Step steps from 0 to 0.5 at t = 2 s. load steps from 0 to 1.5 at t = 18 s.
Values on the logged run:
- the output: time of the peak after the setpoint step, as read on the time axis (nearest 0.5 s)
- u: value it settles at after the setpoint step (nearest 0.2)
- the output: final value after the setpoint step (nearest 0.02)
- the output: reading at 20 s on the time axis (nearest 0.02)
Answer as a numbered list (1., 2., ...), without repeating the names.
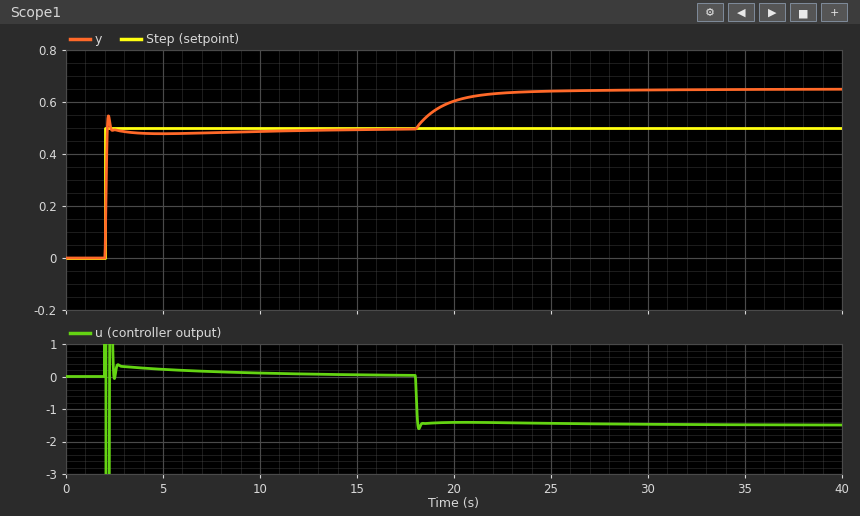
1. 2.0 s
2. 0.0
3. 0.50
4. 0.60
